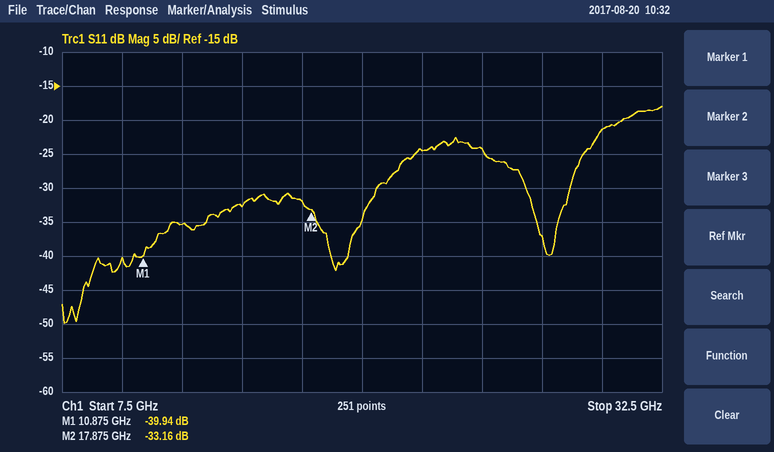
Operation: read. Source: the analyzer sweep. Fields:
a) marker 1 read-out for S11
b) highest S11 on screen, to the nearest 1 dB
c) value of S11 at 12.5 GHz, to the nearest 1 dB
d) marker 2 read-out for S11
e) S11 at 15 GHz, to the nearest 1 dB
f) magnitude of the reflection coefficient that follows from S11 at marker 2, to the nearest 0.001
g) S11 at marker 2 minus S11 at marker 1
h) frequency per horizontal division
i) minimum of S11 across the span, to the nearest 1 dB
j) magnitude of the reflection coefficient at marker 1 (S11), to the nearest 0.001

-39.94 dB
-18 dB
-35 dB
-33.16 dB
-33 dB
0.022
6.78 dB
2.5 GHz
-50 dB
0.010
